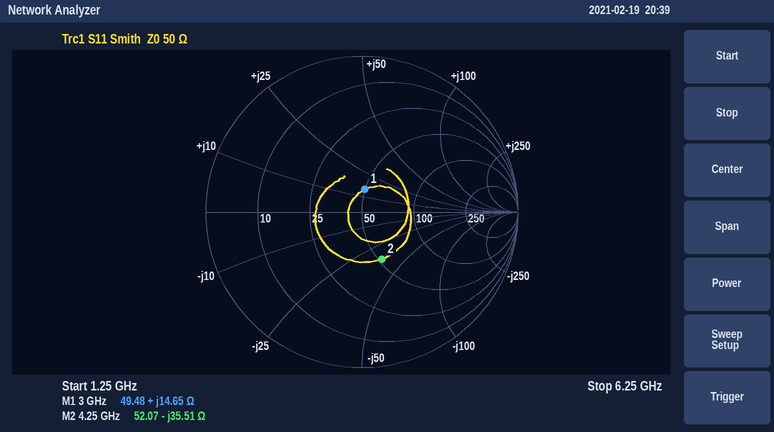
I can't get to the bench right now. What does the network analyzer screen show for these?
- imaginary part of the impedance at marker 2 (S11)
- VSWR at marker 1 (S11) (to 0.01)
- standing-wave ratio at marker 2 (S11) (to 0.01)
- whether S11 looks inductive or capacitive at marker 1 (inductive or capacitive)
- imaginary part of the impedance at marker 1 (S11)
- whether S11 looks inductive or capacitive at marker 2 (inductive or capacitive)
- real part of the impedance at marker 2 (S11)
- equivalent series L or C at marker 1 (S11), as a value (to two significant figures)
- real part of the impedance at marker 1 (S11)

-35.51 Ω
1.34
1.98
inductive
+14.65 Ω
capacitive
52.07 Ω
780 pH
49.48 Ω
